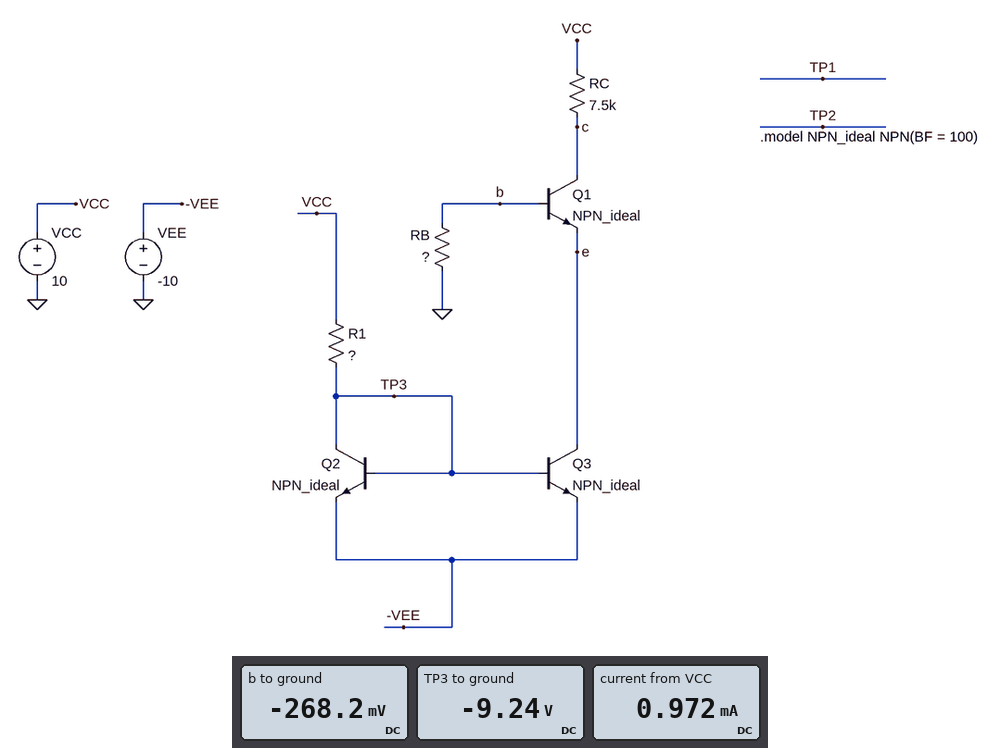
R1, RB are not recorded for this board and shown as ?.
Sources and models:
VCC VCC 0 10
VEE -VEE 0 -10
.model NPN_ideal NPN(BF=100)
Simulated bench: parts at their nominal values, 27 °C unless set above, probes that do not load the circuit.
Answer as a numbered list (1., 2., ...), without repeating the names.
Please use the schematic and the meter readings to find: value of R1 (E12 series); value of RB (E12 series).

1. 39 kΩ
2. 56 kΩ
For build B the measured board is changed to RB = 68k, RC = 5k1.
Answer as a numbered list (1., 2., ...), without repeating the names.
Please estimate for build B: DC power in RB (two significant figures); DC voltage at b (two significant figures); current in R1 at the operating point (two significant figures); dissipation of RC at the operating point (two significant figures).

1. 1.6 µW
2. -330 mV
3. 490 µA
4. 1.2 mW
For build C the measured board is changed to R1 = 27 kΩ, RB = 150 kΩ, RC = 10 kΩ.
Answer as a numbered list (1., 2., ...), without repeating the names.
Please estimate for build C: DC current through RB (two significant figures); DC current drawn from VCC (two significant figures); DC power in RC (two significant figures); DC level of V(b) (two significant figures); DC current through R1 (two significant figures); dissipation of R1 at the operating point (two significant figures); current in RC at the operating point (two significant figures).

1. 6.9 µA
2. 1.4 mA
3. 4.8 mW
4. -1.0 V
5. 710 µA
6. 14 mW
7. 690 µA
